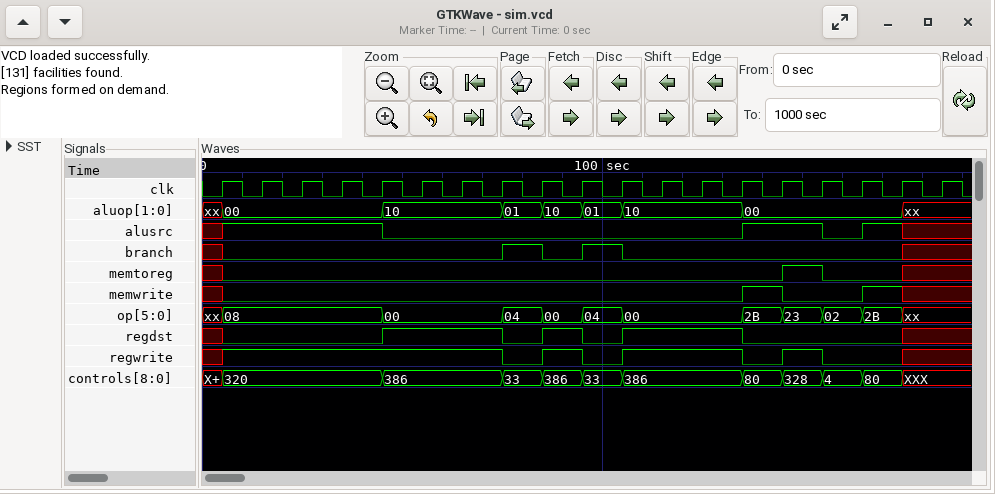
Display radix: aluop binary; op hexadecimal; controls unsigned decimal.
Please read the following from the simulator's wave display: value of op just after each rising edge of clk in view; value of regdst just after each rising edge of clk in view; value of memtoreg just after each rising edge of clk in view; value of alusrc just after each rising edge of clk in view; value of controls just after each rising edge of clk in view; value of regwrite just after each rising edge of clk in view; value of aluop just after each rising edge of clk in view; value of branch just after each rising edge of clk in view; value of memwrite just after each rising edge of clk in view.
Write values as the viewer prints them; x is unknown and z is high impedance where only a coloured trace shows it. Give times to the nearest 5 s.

08, 08, 08, 08, 00, 00, 00, 04, 00, 04, 00, 00, 00, 2B, 23, 02, 2B, xx, xx
0 0 0 0 1 1 1 0 1 0 1 1 1 0 0 0 0 x x
0 0 0 0 0 0 0 0 0 0 0 0 0 0 1 0 0 x x
1 1 1 1 0 0 0 0 0 0 0 0 0 1 1 0 1 x x
320, 320, 320, 320, 386, 386, 386, 33, 386, 33, 386, 386, 386, 80, 328, 4, 80, XXX, XXX
1 1 1 1 1 1 1 0 1 0 1 1 1 0 1 0 0 x x
00, 00, 00, 00, 10, 10, 10, 01, 10, 01, 10, 10, 10, 00, 00, 00, 00, xx, xx
0 0 0 0 0 0 0 1 0 1 0 0 0 0 0 0 0 x x
0 0 0 0 0 0 0 0 0 0 0 0 0 1 0 0 1 x x
